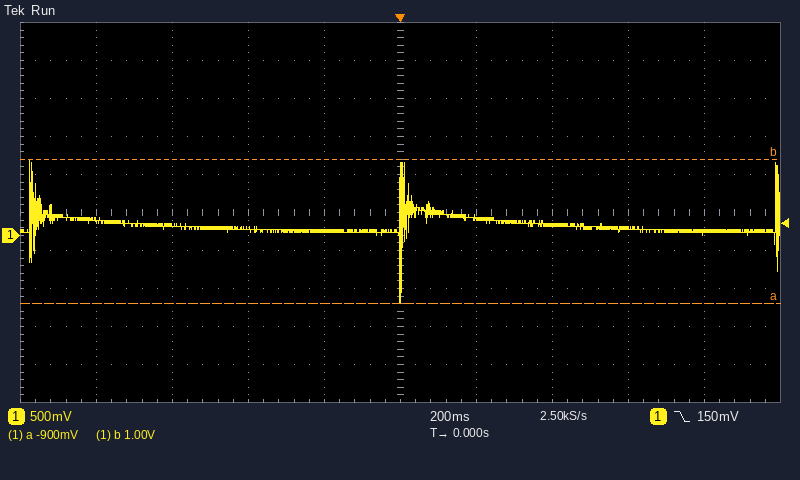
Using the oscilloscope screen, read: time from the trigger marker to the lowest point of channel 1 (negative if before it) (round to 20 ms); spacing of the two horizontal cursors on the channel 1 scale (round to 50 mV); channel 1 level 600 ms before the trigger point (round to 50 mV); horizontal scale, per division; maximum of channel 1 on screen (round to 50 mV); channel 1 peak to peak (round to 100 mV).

0 ms
1.90 V
150 mV
200 ms
1.00 V
1.90 V
